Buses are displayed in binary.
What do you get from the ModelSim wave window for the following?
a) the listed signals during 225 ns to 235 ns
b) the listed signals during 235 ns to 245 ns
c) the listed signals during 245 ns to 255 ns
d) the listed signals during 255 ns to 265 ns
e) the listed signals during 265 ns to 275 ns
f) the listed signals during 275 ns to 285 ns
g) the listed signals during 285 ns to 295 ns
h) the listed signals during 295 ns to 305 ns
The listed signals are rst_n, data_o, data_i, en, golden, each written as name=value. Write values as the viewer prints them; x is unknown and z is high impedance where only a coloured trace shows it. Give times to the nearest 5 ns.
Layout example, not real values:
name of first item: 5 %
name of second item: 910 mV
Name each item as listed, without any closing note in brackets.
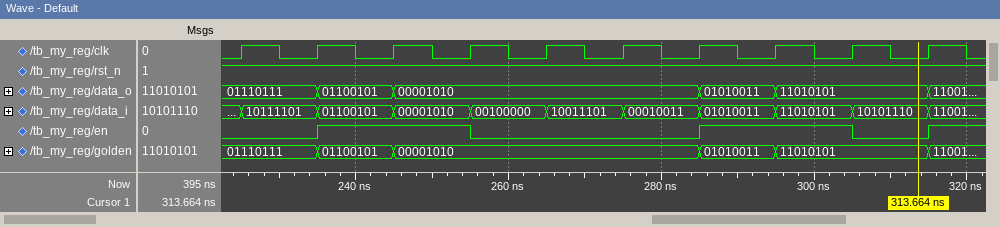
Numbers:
the listed signals during 225 ns to 235 ns: rst_n=1, data_o=01110111, data_i=10111101, en=0, golden=01110111
the listed signals during 235 ns to 245 ns: rst_n=1, data_o=01100101, data_i=01100101, en=1, golden=01100101
the listed signals during 245 ns to 255 ns: rst_n=1, data_o=00001010, data_i=00001010, en=1, golden=00001010
the listed signals during 255 ns to 265 ns: rst_n=1, data_o=00001010, data_i=00100000, en=0, golden=00001010
the listed signals during 265 ns to 275 ns: rst_n=1, data_o=00001010, data_i=10011101, en=0, golden=00001010
the listed signals during 275 ns to 285 ns: rst_n=1, data_o=00001010, data_i=00010011, en=0, golden=00001010
the listed signals during 285 ns to 295 ns: rst_n=1, data_o=01010011, data_i=01010011, en=1, golden=01010011
the listed signals during 295 ns to 305 ns: rst_n=1, data_o=11010101, data_i=11010101, en=1, golden=11010101
